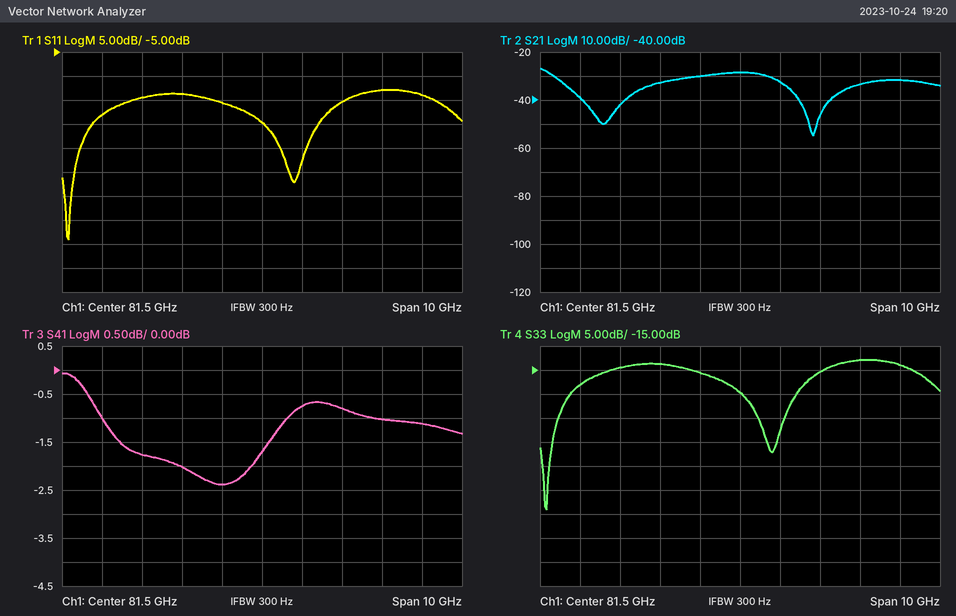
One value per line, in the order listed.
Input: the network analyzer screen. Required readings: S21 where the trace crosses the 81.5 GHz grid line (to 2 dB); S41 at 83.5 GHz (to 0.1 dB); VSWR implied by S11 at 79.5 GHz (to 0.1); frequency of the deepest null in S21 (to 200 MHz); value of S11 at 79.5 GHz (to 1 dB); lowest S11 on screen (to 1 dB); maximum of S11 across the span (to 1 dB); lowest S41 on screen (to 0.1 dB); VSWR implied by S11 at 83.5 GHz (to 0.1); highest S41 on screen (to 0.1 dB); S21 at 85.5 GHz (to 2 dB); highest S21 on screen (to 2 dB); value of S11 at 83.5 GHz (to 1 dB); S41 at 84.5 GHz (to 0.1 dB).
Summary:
-28 dB
-0.8 dB
1.5
83.4 GHz
-14 dB
-44 dB
-13 dB
-2.4 dB
1.4
-0.1 dB
-32 dB
-26 dB
-15 dB
-1.0 dB
